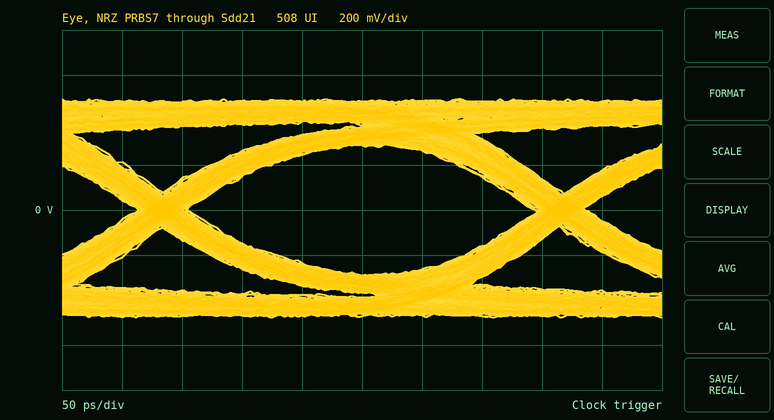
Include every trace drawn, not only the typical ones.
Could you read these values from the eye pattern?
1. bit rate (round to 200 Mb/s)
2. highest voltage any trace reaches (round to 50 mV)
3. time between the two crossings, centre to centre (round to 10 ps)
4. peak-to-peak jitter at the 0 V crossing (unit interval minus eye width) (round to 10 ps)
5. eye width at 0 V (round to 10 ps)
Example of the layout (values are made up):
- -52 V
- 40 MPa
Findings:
- 3.0 Gb/s
- 500 mV
- 330 ps
- 40 ps
- 290 ps
